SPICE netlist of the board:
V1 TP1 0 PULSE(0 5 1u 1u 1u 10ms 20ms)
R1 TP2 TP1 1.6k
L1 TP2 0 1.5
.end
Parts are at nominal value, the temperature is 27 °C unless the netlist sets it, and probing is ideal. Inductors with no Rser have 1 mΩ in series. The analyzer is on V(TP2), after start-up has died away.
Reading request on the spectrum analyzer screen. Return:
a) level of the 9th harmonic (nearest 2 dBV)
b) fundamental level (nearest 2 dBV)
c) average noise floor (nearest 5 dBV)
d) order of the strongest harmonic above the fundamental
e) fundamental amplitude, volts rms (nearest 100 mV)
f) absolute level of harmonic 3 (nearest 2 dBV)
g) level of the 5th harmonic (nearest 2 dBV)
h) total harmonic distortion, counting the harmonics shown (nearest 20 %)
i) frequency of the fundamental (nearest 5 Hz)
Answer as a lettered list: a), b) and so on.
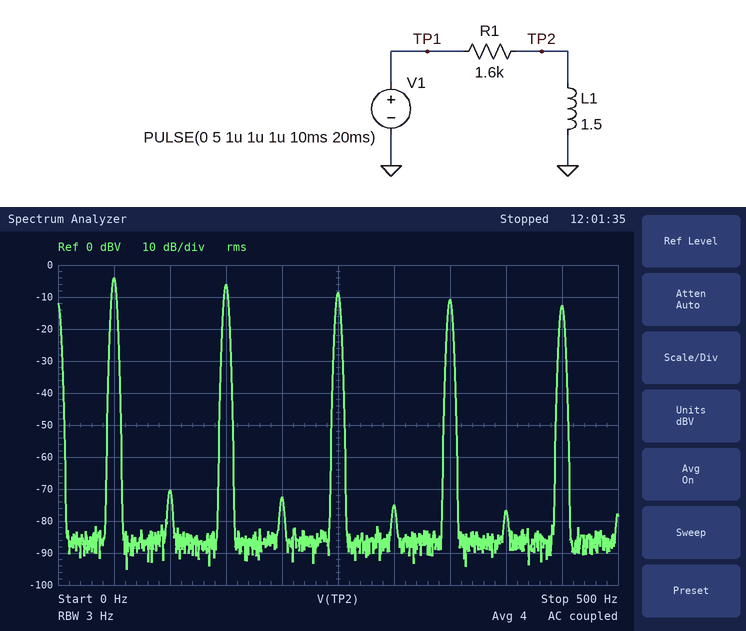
a) -12 dBV
b) -4 dBV
c) -85 dBV
d) 3
e) 600 mV
f) -6 dBV
g) -8 dBV
h) 120 %
i) 50 Hz
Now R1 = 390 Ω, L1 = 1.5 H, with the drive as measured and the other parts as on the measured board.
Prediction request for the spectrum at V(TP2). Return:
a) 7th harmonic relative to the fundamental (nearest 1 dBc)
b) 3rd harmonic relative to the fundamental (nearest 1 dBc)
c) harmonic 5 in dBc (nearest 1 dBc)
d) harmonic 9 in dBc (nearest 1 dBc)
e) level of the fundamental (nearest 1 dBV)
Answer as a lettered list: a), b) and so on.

a) -15 dBc
b) -8 dBc
c) -12 dBc
d) -17 dBc
e) 5 dBV
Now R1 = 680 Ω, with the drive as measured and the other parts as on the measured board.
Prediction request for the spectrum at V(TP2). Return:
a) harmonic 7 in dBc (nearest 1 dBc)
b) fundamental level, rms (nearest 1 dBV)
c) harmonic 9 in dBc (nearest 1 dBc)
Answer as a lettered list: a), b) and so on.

a) -12 dBc
b) 2 dBV
c) -14 dBc
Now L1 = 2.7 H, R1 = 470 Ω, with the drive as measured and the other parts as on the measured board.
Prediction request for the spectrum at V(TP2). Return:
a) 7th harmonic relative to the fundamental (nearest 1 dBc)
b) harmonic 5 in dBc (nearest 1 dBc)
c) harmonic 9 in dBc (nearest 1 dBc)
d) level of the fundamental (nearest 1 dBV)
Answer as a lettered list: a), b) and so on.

a) -16 dBc
b) -13 dBc
c) -18 dBc
d) 6 dBV
